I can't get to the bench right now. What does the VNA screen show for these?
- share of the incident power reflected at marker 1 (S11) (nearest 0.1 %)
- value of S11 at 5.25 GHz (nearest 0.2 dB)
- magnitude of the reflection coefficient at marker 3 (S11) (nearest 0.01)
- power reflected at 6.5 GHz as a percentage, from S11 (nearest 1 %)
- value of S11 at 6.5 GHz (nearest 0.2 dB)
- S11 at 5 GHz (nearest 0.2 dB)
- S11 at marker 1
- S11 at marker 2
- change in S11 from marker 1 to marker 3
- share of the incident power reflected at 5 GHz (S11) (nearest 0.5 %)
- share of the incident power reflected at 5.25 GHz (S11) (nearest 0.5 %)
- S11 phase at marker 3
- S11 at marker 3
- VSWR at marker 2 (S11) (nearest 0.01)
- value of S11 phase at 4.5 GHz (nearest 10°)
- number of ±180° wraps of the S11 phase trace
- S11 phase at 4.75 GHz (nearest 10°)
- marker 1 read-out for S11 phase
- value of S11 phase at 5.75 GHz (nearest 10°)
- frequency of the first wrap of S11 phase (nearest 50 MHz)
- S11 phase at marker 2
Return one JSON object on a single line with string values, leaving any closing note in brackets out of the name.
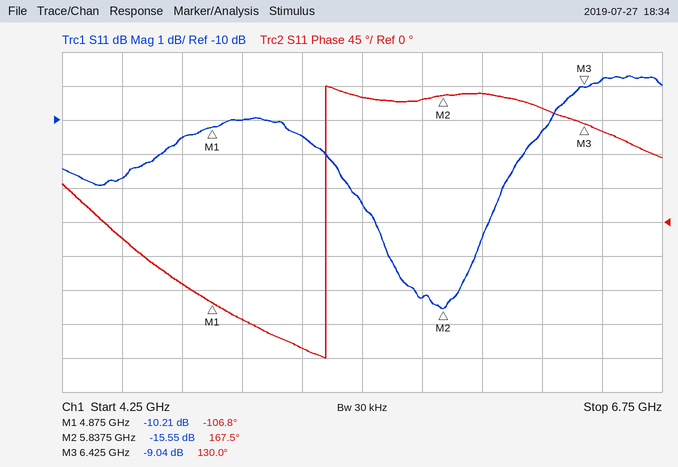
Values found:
{"share of the incident power reflected at marker 1 (S11)": "9.5 %", "value of S11 at 5.25 GHz": "-10.4 dB", "magnitude of the reflection coefficient at marker 3 (S11)": "0.35", "power reflected at 6.5 GHz as a percentage, from S11": "13 %", "value of S11 at 6.5 GHz": "-8.8 dB", "S11 at 5 GHz": "-10.0 dB", "S11 at marker 1": "-10.21 dB", "S11 at marker 2": "-15.55 dB", "change in S11 from marker 1 to marker 3": "1.17 dB", "share of the incident power reflected at 5 GHz (S11)": "10.0 %", "share of the incident power reflected at 5.25 GHz (S11)": "9.0 %", "S11 phase at marker 3": "130.0°", "S11 at marker 3": "-9.04 dB", "VSWR at marker 2 (S11)": "1.40", "value of S11 phase at 4.5 GHz": "-20°", "number of ±180° wraps of the S11 phase trace": "1", "S11 phase at 4.75 GHz": "-80°", "marker 1 read-out for S11 phase": "-106.8°", "value of S11 phase at 5.75 GHz": "160°", "frequency of the first wrap of S11 phase": "5.35 GHz", "S11 phase at marker 2": "167.5°"}
